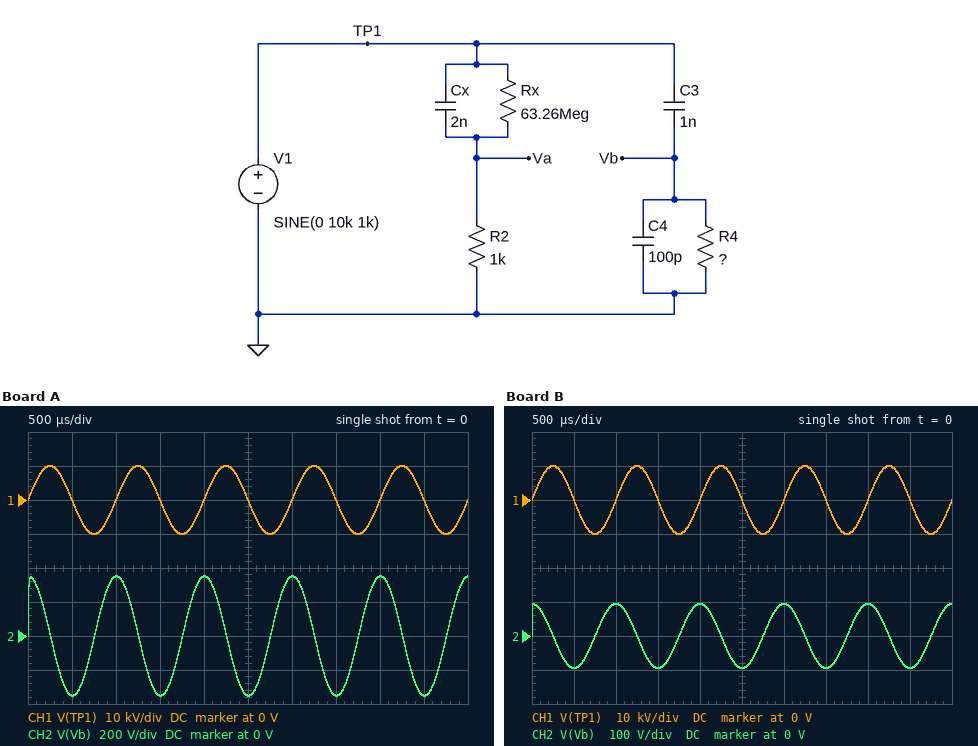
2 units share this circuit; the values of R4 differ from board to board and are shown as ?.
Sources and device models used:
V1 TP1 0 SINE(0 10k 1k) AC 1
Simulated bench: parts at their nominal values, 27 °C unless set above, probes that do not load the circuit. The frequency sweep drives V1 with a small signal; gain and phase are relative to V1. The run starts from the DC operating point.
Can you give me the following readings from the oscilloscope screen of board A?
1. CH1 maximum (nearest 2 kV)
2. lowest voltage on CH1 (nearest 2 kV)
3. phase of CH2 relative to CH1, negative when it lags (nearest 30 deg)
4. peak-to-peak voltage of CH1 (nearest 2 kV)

10 kV
-10 kV
90 deg
20 kV
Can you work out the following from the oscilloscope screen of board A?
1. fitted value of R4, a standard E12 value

5.6 kΩ
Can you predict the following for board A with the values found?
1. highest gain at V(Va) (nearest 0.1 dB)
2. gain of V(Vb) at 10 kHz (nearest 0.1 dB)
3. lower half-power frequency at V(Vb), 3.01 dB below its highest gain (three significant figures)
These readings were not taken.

0 dB
-9.7 dB
25.8 kHz
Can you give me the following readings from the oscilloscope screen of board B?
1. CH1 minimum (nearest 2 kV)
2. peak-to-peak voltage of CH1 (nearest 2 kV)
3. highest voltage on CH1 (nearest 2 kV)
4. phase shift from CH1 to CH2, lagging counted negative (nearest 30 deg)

-10 kV
20 kV
10 kV
90 deg
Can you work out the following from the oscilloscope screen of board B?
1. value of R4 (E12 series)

1.5 kΩ
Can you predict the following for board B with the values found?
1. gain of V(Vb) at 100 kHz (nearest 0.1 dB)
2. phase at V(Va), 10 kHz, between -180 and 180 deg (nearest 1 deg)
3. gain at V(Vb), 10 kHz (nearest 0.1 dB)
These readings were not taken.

-3.7 dB
83 deg
-20.6 dB
